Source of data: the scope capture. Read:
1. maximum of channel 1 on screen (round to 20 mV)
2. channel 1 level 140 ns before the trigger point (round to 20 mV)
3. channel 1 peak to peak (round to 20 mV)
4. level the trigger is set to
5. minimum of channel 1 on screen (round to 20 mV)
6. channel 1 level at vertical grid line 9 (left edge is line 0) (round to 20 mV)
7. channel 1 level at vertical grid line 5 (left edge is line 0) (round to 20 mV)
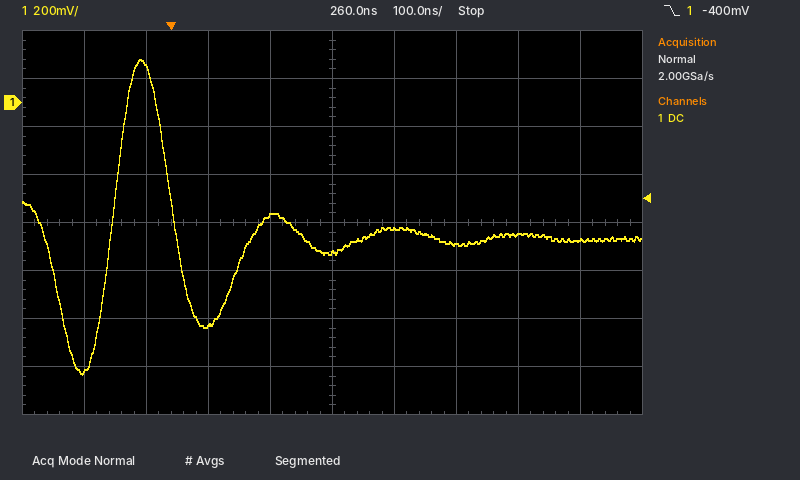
180 mV
-1.12 V
1.32 V
-400 mV
-1.14 V
-580 mV
-620 mV
